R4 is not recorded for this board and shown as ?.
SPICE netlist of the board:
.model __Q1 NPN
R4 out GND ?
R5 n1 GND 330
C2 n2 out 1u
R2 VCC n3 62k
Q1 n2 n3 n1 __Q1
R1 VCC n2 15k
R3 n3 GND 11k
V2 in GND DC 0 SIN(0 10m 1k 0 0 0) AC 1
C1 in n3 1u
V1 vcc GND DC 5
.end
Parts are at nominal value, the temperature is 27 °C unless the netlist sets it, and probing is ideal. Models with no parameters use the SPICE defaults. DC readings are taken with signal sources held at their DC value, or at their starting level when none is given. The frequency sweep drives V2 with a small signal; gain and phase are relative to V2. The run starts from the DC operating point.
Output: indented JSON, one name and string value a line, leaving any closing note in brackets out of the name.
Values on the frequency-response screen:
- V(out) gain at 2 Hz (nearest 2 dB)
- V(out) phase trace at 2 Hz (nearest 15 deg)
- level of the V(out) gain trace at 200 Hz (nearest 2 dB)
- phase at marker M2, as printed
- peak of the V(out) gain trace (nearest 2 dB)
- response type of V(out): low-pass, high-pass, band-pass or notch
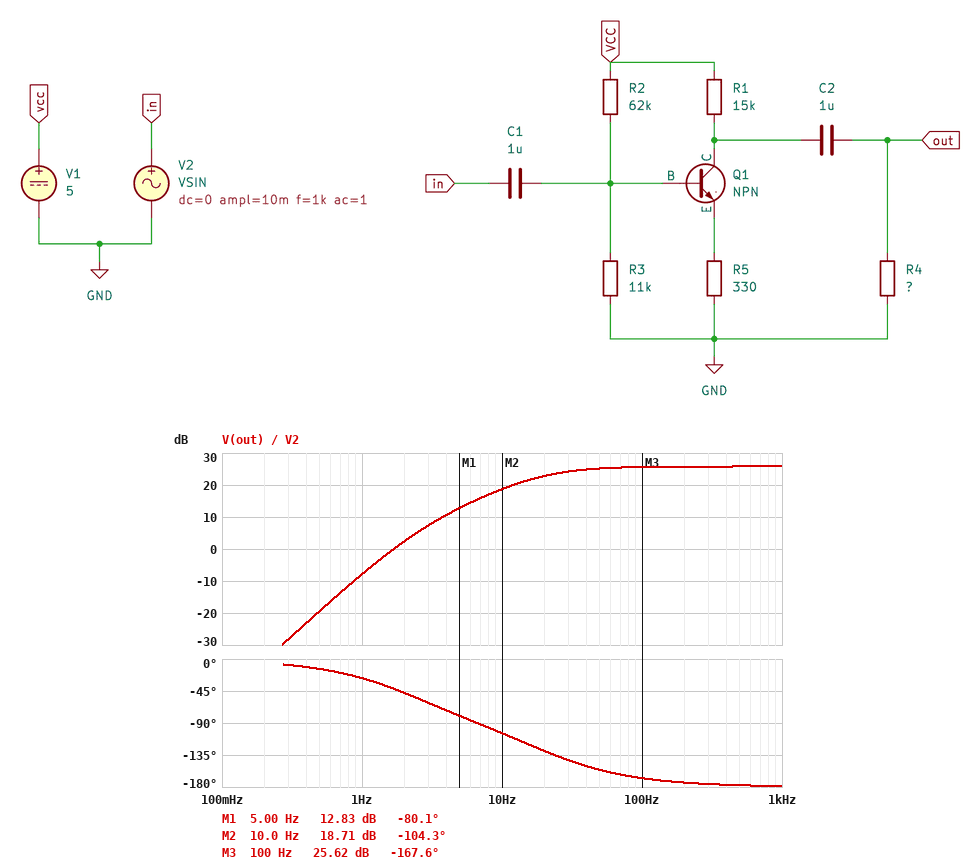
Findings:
{
  "V(out) gain at 2 Hz": "2 dB",
  "V(out) phase trace at 2 Hz": "-45 deg",
  "level of the V(out) gain trace at 200 Hz": "26 dB",
  "phase at marker M2, as printed": "-104.3 deg",
  "peak of the V(out) gain trace": "26 dB",
  "response type of V(out): low-pass, high-pass, band-pass or notch": "high-pass"
}
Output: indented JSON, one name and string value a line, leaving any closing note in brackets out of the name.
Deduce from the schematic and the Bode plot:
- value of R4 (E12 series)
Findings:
{
  "value of R4": "56 kΩ"
}
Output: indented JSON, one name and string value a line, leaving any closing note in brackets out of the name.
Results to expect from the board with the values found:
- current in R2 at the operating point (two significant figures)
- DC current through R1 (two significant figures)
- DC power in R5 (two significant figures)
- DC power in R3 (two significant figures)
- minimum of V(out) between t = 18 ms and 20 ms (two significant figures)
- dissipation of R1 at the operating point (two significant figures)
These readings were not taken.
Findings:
{
  "current in R2 at the operating point": "69 µA",
  "DC current through R1": "94 µA",
  "DC power in R5": "3.0 µW",
  "DC power in R3": "50 µW",
  "minimum of V(out) between t = 18 ms and 20 ms": "-200 mV",
  "dissipation of R1 at the operating point": "130 µW"
}
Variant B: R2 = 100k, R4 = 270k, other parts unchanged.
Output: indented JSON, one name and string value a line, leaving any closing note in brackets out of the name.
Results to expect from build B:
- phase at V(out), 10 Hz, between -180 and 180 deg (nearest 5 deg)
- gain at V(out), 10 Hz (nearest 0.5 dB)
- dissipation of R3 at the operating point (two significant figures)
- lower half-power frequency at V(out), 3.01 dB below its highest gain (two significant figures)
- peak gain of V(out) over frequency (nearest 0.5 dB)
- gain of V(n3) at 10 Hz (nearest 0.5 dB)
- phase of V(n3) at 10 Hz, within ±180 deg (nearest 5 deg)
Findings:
{
  "phase at V(out), 10 Hz, between -180 and 180 deg": "-120 deg",
  "gain at V(out), 10 Hz": "-44.5 dB",
  "dissipation of R3 at the operating point": "22 µW",
  "lower half-power frequency at V(out), 3.01 dB below its highest gain": "16 Hz",
  "peak gain of V(out) over frequency": "-39.0 dB",
  "gain of V(n3) at 10 Hz": "-5.5 dB",
  "phase of V(n3) at 10 Hz, within ±180 deg": "60 deg"
}
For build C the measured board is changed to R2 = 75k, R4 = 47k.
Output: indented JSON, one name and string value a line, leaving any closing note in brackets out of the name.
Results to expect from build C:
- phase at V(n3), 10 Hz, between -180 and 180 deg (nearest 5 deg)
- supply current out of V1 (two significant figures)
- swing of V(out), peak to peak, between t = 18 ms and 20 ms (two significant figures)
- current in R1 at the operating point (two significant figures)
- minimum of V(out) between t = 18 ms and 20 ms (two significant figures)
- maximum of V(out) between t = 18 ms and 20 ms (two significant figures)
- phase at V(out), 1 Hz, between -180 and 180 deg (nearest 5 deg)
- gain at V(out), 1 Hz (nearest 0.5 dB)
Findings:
{
  "phase at V(n3), 10 Hz, between -180 and 180 deg": "60 deg",
  "supply current out of V1": "63 µA",
  "swing of V(out), peak to peak, between t = 18 ms and 20 ms": "42 mV",
  "current in R1 at the operating point": "5.0 µA",
  "minimum of V(out) between t = 18 ms and 20 ms": "-24 mV",
  "maximum of V(out) between t = 18 ms and 20 ms": "18 mV",
  "phase at V(out), 1 Hz, between -180 and 180 deg": "-25 deg",
  "gain at V(out), 1 Hz": "-27.0 dB"
}
